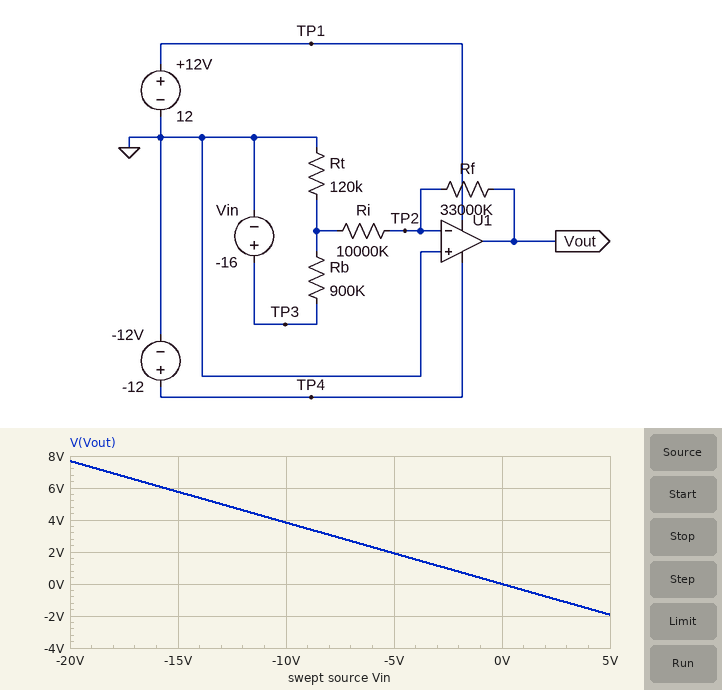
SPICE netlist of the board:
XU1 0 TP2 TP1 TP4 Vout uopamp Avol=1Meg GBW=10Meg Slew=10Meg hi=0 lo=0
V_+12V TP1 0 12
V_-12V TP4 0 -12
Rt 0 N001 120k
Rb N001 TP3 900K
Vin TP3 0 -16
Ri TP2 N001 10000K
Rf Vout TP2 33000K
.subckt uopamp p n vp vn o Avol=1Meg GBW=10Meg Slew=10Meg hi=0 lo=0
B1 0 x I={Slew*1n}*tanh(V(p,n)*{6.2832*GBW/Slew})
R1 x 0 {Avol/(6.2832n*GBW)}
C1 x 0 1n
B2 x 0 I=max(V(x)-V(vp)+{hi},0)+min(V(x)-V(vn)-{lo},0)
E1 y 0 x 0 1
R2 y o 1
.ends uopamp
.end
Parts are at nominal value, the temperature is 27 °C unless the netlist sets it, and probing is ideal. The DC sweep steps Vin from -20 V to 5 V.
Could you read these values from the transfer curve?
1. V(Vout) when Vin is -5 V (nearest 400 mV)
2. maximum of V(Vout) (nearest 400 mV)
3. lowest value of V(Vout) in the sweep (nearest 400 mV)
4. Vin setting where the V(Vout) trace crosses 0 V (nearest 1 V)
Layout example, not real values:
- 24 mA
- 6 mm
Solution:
- 2.0 V
- 7.6 V
- -2.0 V
- 0 V
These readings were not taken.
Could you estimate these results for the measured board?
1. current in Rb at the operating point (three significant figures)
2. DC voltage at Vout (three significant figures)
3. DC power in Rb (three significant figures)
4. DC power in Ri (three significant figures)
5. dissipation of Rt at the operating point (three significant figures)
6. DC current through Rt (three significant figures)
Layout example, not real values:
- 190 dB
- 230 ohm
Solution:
- 15.7 µA
- 6.15 V
- 222 µW
- 347 nW
- 28.9 µW
- 15.5 µA
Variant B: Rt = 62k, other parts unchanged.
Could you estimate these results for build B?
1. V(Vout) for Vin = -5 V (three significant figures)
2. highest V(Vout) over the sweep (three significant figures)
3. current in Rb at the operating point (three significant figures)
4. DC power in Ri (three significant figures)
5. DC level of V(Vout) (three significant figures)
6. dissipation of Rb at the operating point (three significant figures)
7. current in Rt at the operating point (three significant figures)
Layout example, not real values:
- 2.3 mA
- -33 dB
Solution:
- 1.06 V
- 4.23 V
- 16.6 µA
- 105 nW
- 3.38 V
- 249 µW
- 16.5 µA
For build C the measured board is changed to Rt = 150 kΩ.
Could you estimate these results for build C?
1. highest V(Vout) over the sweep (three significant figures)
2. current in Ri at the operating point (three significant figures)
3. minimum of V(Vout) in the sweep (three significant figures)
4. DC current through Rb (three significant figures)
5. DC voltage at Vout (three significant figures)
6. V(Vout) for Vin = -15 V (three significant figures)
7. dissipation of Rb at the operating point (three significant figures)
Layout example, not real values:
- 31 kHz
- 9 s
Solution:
- 9.31 V
- 226 nA
- -2.33 V
- 15.3 µA
- 7.45 V
- 6.98 V
- 210 µW
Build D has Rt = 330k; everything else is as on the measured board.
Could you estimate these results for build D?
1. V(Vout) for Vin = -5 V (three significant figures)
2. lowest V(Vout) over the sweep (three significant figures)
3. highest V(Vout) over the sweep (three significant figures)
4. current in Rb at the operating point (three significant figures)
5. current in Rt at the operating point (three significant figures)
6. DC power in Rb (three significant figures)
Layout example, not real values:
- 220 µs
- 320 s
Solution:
- 4.32 V
- -4.32 V
- 12.0 V
- 13.1 µA
- 12.7 µA
- 155 µW
